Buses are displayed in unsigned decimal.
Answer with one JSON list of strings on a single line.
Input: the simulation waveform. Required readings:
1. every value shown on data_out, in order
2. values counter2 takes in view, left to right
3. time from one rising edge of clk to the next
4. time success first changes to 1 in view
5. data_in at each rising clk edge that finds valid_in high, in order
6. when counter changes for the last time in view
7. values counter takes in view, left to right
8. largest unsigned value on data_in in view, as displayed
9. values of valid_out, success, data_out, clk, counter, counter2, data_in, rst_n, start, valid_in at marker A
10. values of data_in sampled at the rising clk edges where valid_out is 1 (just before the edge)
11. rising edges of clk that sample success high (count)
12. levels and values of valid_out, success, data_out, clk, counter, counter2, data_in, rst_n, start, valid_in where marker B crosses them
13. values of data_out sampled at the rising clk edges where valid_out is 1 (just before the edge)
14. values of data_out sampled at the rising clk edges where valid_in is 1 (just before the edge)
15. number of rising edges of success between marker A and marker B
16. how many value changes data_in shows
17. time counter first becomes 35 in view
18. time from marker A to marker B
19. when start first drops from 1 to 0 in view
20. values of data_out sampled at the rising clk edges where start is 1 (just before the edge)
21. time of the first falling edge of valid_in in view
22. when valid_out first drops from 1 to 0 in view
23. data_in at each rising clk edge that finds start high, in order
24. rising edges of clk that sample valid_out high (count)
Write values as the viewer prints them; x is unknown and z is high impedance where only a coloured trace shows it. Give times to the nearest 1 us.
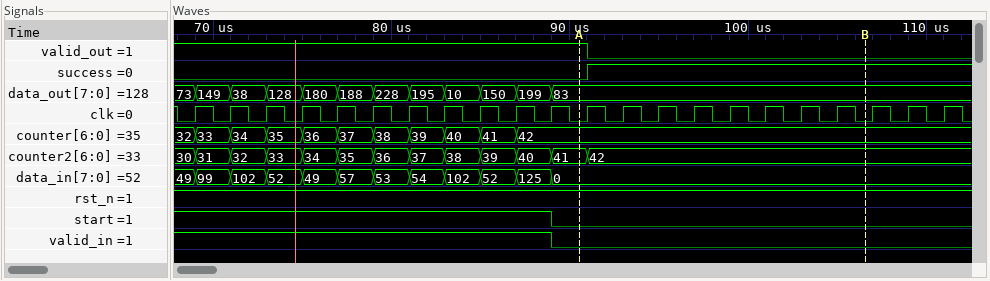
["73, 149, 38, 128, 180, 188, 228, 195, 10, 150, 199, 83", "30, 31, 32, 33, 34, 35, 36, 37, 38, 39, 40, 41, 42", "2 us", "91 us", "49, 99, 102, 52, 49, 57, 53, 54, 102, 52, 125", "87 us", "32, 33, 34, 35, 36, 37, 38, 39, 40, 41, 42", "125", "valid_out=1, success=0, data_out=83, clk=0, counter=42, counter2=41, data_in=0, rst_n=1, start=0, valid_in=0", "49, 99, 102, 52, 49, 57, 53, 54, 102, 52, 125, 0", "10", "valid_out=0, success=1, data_out=83, clk=0, counter=42, counter2=42, data_in=0, rst_n=1, start=0, valid_in=0", "73, 149, 38, 128, 180, 188, 228, 195, 10, 150, 199, 83", "73, 149, 38, 128, 180, 188, 228, 195, 10, 150, 199", "1", "11", "73 us", "16 us", "89 us", "73, 149, 38, 128, 180, 188, 228, 195, 10, 150, 199", "89 us", "91 us", "49, 99, 102, 52, 49, 57, 53, 54, 102, 52, 125", "12"]
